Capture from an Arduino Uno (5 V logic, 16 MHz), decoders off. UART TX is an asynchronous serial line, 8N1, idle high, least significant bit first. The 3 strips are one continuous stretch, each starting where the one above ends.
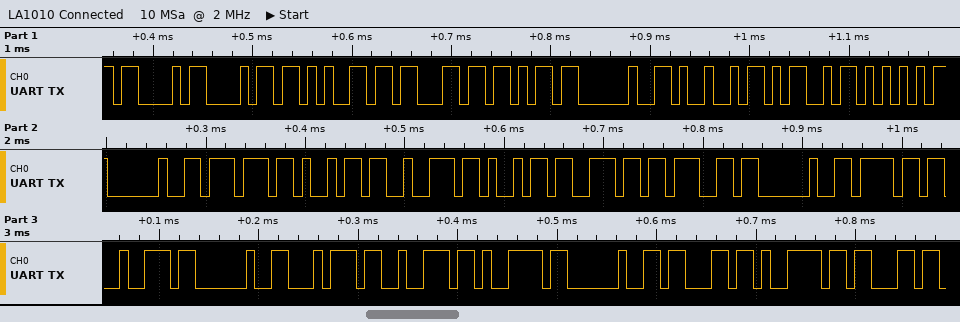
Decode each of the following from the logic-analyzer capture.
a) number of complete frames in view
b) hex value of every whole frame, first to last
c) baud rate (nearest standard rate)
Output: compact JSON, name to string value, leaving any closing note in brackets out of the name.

{"number of complete frames in view": "27", "hex value of every whole frame, first to last": "43 68 65 63 6B 20 49 4D 55 20 77 69 72 69 6E 67 20 6F 72 20 74 72 79 20 63 79 63", "baud rate": "115200 baud"}
